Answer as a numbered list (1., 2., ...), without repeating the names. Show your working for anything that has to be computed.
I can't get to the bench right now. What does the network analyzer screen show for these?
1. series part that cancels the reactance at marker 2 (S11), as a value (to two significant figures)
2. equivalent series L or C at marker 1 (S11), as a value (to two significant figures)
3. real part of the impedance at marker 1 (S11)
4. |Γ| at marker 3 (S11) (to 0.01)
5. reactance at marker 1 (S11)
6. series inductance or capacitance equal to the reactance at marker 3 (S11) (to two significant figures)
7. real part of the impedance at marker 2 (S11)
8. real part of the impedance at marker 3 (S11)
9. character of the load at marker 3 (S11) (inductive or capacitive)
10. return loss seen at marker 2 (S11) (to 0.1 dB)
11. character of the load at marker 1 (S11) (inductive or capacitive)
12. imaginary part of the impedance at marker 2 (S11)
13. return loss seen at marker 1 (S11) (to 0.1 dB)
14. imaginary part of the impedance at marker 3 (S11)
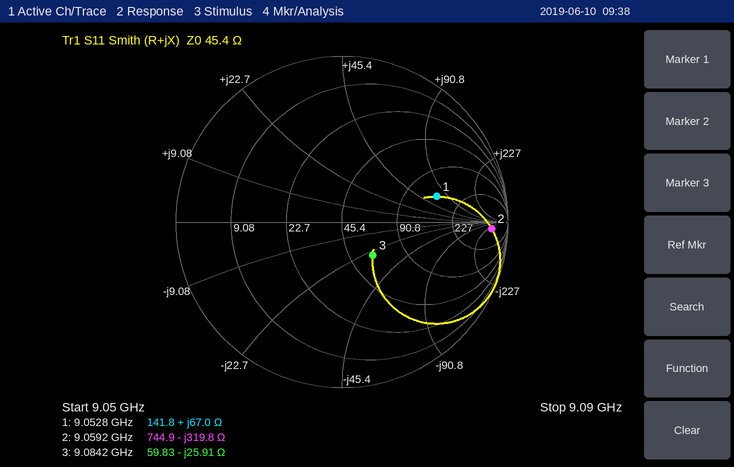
1. L = 319.8 Ω/(2π × 9.0592 GHz) ≈ 5.6 nH
2. L = 67 Ω/(2π × 9.0528 GHz) ≈ 1.2 nH
3. 141.8 Ω
4. 0.27
5. +67.0 Ω
6. C = 1/(2π × 9.0842 GHz × 25.91 Ω) ≈ 676 fF, so 680 fF to two significant figures
7. 744.9 Ω
8. 59.83 Ω
9. capacitive
10. 0.9 dB
11. inductive
12. -319.8 Ω
13. 4.6 dB
14. -25.91 Ω
